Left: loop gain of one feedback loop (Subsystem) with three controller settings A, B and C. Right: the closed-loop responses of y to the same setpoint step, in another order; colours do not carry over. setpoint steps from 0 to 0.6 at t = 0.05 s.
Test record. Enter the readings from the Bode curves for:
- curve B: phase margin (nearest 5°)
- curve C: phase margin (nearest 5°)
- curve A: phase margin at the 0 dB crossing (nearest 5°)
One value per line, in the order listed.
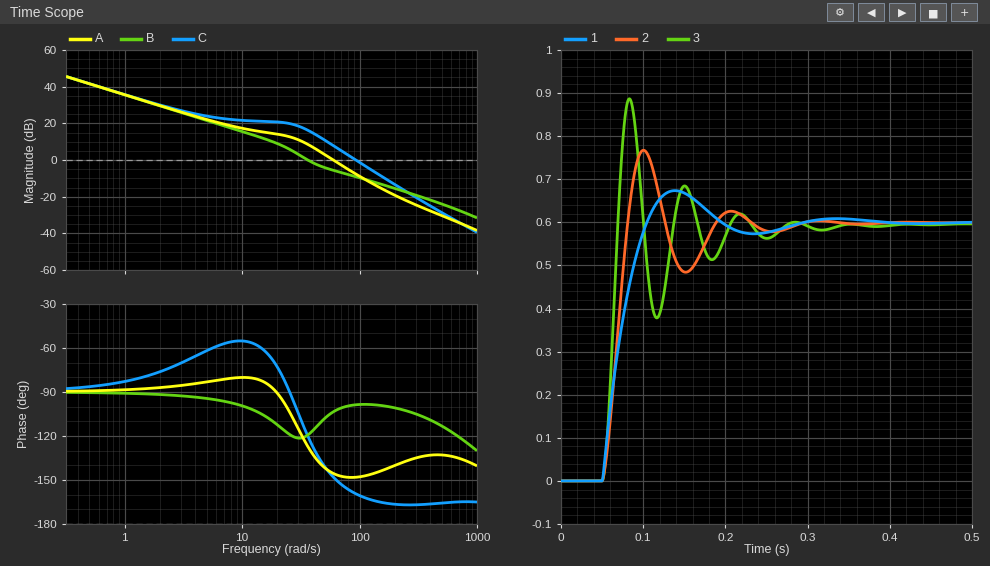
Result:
60°
20°
35°
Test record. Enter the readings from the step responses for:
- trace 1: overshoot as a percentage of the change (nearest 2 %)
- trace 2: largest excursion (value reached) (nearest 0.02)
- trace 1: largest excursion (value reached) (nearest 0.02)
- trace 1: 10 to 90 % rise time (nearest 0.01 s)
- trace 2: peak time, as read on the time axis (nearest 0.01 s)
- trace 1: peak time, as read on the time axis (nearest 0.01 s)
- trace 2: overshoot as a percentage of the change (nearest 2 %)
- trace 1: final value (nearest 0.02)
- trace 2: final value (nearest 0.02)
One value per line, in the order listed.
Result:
12 %
0.76
0.68
0.04 s
0.10 s
0.14 s
28 %
0.60
0.60
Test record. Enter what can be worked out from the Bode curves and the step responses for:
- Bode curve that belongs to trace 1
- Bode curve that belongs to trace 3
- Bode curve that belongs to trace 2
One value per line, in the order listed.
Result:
B
C
A
